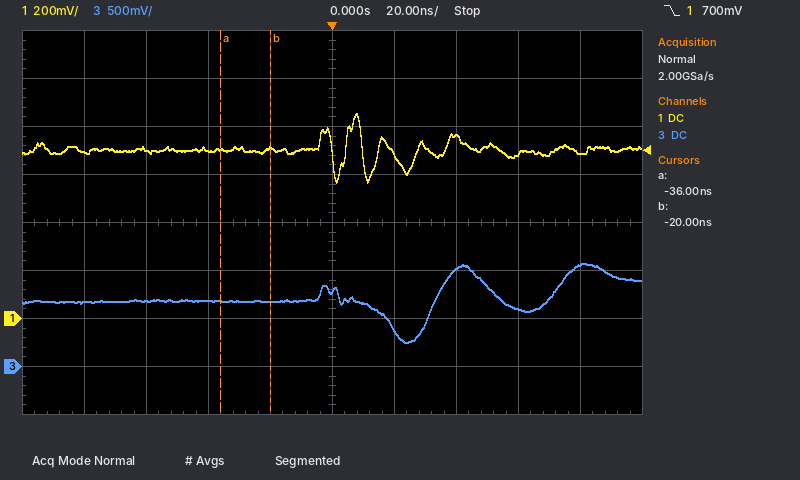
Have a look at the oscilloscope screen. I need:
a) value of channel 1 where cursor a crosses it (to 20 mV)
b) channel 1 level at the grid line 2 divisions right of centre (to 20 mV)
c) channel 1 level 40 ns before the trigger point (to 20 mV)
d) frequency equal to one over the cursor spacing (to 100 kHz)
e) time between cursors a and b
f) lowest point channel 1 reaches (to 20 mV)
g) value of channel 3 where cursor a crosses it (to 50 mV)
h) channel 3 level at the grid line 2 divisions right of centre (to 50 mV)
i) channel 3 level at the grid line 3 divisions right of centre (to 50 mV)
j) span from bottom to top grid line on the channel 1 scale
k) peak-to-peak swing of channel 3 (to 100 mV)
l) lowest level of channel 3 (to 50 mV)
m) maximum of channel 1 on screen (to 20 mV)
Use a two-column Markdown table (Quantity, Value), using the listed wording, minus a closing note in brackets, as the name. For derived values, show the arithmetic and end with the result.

| Quantity | Value |
|---|---|
| value of channel 1 where cursor a crosses it | 700 mV |
| channel 1 level at the grid line 2 divisions right of centre | 760 mV |
| channel 1 level 40 ns before the trigger point | 700 mV |
| frequency equal to one over the cursor spacing | 1 / 16 ns ≈ 62.5 MHz |
| time between cursors a and b | -20 ns − (-36 ns) = 16 ns |
| lowest point channel 1 reaches | 560 mV |
| value of channel 3 where cursor a crosses it | 700 mV |
| channel 3 level at the grid line 2 divisions right of centre | 1.00 V |
| channel 3 level at the grid line 3 divisions right of centre | 600 mV |
| span from bottom to top grid line on the channel 1 scale | 1.6 V |
| peak-to-peak swing of channel 3 | 800 mV |
| lowest level of channel 3 | 250 mV |
| maximum of channel 1 on screen | 860 mV |
